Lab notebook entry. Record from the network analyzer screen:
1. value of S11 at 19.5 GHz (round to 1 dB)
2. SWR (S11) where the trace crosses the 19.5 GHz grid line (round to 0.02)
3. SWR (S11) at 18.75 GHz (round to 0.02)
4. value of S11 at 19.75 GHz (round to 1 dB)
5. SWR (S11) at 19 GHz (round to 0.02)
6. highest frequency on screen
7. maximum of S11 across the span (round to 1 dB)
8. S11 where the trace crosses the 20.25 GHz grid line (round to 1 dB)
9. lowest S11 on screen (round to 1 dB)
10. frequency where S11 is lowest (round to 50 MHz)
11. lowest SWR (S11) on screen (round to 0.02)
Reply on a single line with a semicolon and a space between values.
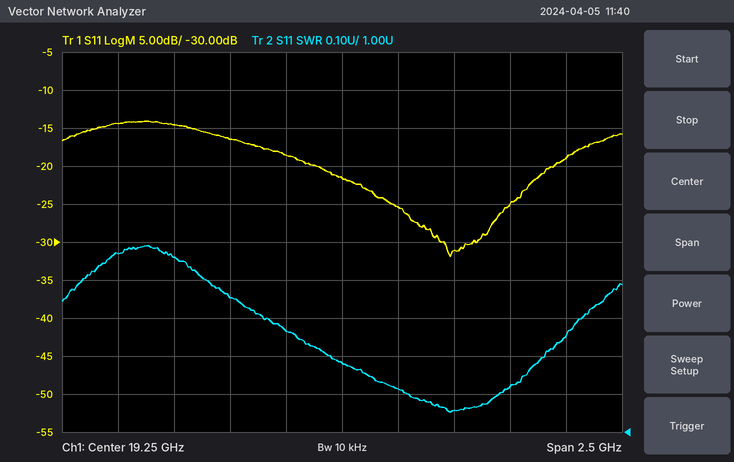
-25 dB; 1.12; 1.36; -31 dB; 1.26; 20.5 GHz; -14 dB; -19 dB; -32 dB; 19.75 GHz; 1.06
